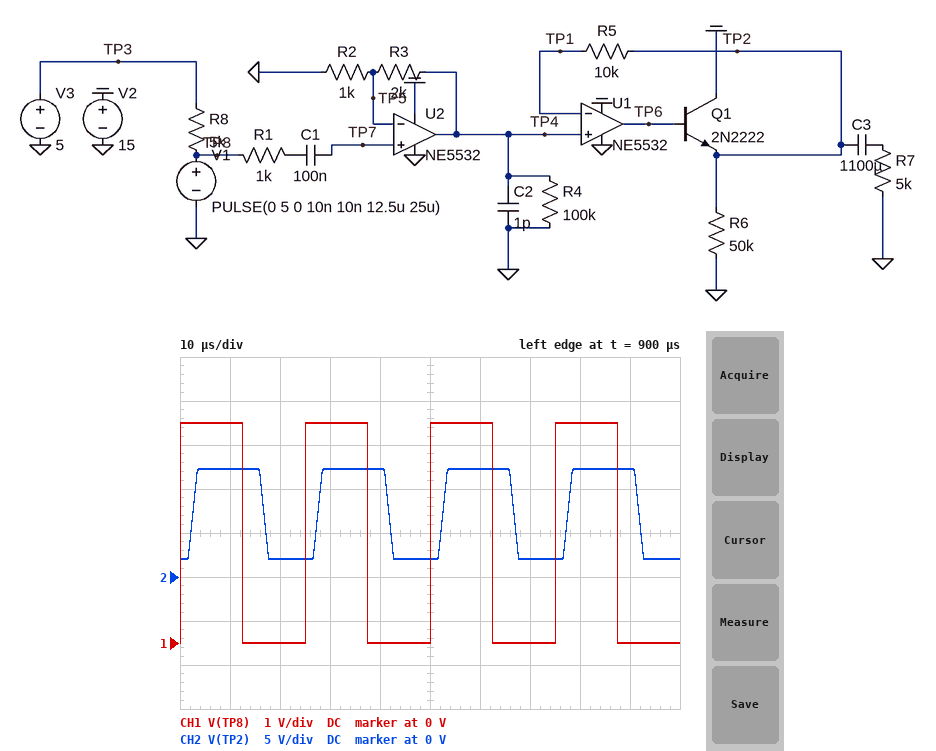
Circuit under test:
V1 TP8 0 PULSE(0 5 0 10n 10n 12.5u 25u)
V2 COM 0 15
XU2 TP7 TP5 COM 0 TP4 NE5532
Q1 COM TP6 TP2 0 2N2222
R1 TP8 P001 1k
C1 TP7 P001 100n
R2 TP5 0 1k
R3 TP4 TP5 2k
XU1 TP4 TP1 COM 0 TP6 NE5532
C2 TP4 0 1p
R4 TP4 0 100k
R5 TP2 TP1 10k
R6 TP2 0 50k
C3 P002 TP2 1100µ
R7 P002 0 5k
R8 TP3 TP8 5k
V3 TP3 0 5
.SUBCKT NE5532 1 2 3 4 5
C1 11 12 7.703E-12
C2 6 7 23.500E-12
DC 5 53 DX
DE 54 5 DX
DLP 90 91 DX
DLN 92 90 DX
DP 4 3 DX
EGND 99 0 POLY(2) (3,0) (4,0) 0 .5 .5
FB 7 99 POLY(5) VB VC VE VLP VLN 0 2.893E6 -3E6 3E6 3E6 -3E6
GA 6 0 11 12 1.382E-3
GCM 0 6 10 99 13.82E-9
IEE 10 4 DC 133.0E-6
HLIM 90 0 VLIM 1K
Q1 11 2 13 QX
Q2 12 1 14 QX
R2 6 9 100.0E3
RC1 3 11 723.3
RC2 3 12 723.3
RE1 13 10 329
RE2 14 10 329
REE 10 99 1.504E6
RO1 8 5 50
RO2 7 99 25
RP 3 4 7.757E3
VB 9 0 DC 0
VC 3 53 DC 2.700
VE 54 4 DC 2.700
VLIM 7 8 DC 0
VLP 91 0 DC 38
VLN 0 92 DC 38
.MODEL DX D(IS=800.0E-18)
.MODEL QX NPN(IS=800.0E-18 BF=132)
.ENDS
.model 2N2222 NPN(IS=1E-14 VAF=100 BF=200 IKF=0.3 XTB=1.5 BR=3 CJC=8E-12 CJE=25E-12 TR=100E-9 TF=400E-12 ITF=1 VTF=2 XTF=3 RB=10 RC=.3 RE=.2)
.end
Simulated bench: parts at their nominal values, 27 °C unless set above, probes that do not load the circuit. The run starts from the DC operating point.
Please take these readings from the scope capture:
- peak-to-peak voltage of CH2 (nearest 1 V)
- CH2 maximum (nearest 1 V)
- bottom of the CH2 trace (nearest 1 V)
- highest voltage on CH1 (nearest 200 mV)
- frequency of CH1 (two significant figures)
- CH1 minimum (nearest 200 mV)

10 V
12 V
2 V
5.0 V
40 kHz
0 V
